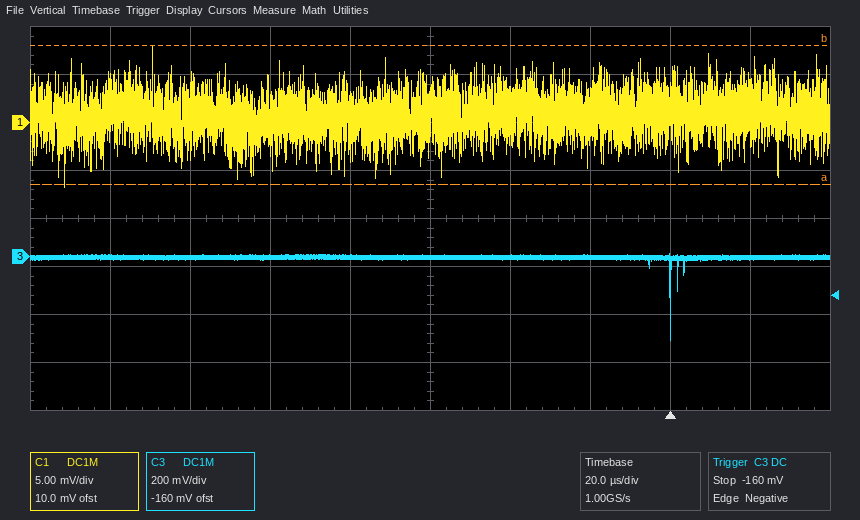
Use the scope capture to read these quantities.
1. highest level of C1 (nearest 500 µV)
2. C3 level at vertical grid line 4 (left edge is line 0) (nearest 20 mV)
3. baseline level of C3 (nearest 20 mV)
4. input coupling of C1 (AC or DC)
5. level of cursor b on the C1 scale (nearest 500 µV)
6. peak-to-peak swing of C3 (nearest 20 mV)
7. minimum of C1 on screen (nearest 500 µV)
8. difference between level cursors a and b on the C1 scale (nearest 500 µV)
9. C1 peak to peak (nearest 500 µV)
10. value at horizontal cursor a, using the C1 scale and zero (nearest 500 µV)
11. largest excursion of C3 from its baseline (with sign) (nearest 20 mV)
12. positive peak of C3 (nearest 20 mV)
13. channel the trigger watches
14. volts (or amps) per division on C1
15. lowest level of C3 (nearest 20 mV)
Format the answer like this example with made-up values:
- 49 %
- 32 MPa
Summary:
- 8.0 mV
- 0 mV
- 0 mV
- DC
- 8.0 mV
- 360 mV
- -6.5 mV
- 14.5 mV
- 14.5 mV
- -6.5 mV
- -340 mV
- 20 mV
- C3
- 5 mV
- -340 mV
